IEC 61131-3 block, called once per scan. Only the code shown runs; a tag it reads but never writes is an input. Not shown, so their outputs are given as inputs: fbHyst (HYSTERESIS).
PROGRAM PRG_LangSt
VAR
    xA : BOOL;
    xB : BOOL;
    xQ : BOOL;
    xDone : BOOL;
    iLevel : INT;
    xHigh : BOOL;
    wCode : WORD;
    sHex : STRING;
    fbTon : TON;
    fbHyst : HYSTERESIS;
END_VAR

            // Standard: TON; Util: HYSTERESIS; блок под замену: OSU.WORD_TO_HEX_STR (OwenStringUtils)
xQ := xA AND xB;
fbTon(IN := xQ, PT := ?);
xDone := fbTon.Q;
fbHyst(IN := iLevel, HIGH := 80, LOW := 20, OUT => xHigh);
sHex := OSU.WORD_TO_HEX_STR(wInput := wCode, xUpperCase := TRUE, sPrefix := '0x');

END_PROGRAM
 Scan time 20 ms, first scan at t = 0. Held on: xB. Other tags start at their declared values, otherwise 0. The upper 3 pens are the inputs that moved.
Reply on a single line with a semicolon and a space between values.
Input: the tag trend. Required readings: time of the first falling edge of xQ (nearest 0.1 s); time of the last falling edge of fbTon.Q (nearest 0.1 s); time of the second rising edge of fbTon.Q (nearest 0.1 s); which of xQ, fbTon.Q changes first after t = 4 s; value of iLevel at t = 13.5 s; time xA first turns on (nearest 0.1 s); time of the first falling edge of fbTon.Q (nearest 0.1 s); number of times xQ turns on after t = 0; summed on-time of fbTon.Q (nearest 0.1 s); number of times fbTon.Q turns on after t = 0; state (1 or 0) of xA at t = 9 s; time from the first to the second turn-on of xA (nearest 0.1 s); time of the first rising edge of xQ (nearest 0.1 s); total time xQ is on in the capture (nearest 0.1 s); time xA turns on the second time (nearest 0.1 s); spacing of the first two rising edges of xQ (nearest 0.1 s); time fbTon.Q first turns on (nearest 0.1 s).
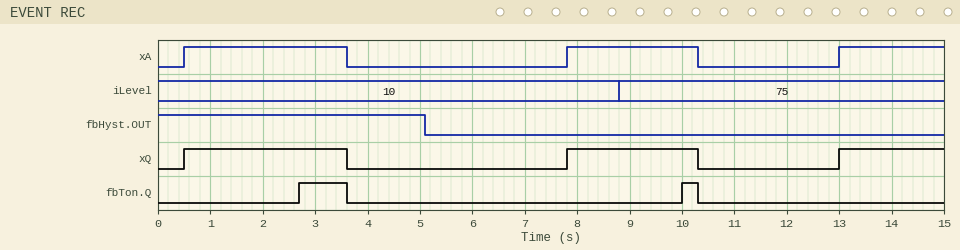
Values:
3.6 s; 10.3 s; 10.0 s; xQ; 75; 0.5 s; 3.6 s; 3; 1.2 s; 2; 1; 7.3 s; 0.5 s; 7.6 s; 7.8 s; 7.3 s; 2.7 s
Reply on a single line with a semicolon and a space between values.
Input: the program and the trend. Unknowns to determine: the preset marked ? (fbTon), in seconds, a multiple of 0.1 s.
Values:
2.2 s
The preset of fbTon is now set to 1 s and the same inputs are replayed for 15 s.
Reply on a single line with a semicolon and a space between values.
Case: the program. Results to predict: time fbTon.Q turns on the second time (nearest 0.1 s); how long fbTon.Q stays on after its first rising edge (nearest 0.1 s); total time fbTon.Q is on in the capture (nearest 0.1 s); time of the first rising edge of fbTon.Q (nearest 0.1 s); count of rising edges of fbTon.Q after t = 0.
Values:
8.8 s; 2.1 s; 4.6 s; 1.5 s; 3
